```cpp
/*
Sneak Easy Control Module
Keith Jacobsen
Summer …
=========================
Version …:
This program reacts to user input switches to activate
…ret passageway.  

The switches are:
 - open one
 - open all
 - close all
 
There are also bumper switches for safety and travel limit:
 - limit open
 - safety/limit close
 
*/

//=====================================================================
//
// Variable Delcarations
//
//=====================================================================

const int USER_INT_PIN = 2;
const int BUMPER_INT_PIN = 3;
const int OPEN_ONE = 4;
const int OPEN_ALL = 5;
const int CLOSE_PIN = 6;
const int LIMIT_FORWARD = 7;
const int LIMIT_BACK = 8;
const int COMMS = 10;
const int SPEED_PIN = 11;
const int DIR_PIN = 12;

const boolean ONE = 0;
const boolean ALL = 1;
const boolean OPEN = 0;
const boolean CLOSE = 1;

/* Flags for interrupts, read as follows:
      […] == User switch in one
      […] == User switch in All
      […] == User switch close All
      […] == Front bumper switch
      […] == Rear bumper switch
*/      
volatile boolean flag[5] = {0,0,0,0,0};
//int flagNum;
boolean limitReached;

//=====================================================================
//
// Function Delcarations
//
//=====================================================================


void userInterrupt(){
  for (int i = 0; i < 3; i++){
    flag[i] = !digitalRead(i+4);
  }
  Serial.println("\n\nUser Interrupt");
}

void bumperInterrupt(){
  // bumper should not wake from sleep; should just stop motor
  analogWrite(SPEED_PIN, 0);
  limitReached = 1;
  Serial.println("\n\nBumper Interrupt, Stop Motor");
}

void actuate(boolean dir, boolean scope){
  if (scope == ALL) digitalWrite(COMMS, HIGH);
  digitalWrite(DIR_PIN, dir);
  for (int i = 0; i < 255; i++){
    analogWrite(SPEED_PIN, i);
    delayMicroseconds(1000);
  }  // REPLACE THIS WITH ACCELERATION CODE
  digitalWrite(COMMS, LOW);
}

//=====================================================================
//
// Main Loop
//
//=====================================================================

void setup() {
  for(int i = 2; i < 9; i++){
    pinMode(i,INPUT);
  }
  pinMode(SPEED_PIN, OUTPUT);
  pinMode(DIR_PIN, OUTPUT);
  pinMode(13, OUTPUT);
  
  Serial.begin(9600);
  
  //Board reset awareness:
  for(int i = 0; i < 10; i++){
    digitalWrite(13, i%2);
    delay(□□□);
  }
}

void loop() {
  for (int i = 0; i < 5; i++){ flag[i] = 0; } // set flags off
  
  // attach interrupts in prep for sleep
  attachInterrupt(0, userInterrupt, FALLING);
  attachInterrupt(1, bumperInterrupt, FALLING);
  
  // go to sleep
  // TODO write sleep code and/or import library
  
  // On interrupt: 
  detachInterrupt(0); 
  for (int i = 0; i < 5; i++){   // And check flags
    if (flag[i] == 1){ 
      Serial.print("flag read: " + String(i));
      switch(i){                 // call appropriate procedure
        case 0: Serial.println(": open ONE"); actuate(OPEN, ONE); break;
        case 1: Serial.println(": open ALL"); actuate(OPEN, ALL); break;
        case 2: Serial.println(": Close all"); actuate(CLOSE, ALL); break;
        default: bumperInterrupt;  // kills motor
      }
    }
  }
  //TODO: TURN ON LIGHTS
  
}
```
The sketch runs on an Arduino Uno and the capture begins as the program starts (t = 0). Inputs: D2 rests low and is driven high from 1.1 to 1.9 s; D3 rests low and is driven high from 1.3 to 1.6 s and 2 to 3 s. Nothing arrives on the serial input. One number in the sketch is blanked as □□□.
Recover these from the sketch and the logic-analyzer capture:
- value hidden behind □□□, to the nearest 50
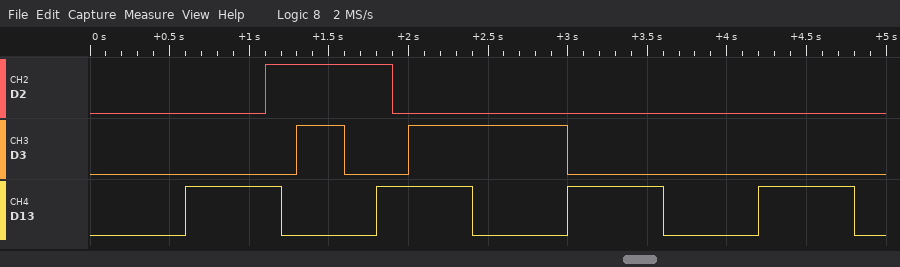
600
